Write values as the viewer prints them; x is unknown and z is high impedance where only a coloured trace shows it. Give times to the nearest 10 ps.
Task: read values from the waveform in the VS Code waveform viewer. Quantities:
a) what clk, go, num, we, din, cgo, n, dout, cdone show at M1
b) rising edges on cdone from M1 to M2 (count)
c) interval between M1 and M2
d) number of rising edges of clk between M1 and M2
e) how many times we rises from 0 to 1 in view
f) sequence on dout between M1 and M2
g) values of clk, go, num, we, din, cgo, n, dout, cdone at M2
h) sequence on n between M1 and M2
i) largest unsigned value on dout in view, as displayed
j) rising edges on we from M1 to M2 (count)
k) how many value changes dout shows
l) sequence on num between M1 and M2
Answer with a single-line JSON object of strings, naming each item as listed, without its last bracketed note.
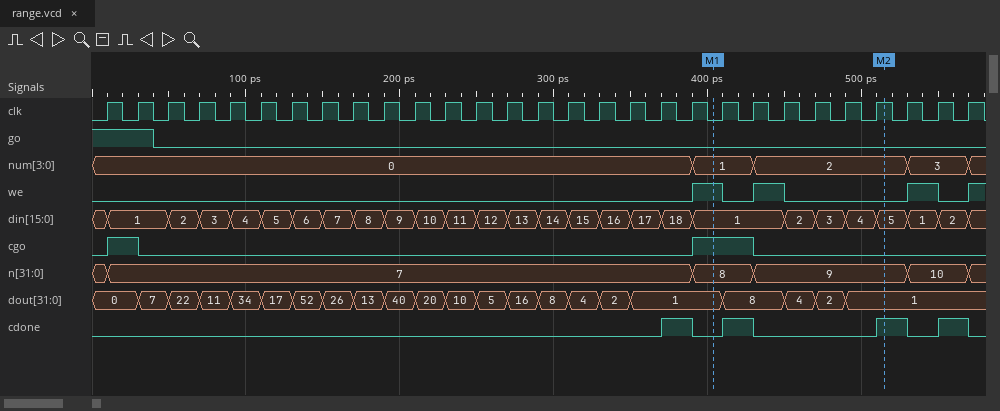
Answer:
{"what clk, go, num, we, din, cgo, n, dout, cdone show at M1": "clk=0, go=0, num=1, we=1, din=1, cgo=1, n=8, dout=1, cdone=0", "rising edges on cdone from M1 to M2": "2", "interval between M1 and M2": "110 ps", "number of rising edges of clk between M1 and M2": "6", "how many times we rises from 0 to 1 in view": "4", "sequence on dout between M1 and M2": "1, 8, 4, 2, 1", "values of clk, go, num, we, din, cgo, n, dout, cdone at M2": "clk=1, go=0, num=2, we=0, din=5, cgo=0, n=9, dout=1, cdone=1", "sequence on n between M1 and M2": "8, 9", "largest unsigned value on dout in view, as displayed": "52", "rising edges on we from M1 to M2": "1", "how many value changes dout shows": "21", "sequence on num between M1 and M2": "1, 2"}
